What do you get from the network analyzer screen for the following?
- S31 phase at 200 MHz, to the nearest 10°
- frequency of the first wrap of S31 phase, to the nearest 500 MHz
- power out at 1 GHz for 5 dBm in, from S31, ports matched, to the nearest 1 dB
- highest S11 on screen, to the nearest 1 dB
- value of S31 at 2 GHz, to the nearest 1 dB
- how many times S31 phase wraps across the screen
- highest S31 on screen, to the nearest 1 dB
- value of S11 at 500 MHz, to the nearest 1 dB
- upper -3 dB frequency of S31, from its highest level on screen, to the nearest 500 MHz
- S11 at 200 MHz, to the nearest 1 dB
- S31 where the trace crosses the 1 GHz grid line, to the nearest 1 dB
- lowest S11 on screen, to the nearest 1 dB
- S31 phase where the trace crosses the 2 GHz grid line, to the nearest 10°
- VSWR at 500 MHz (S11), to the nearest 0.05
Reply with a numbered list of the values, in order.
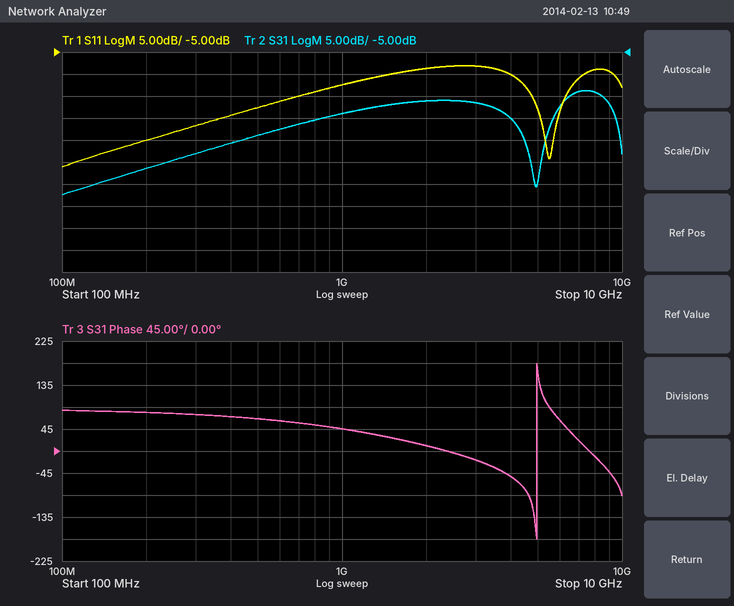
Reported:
1. 80°
2. 5.0 GHz
3. -14 dBm
4. -8 dB
5. -16 dB
6. 1
7. -14 dB
8. -18 dB
9. 9.0 GHz
10. -25 dB
11. -19 dB
12. -31 dB
13. 10°
14. 1.30
